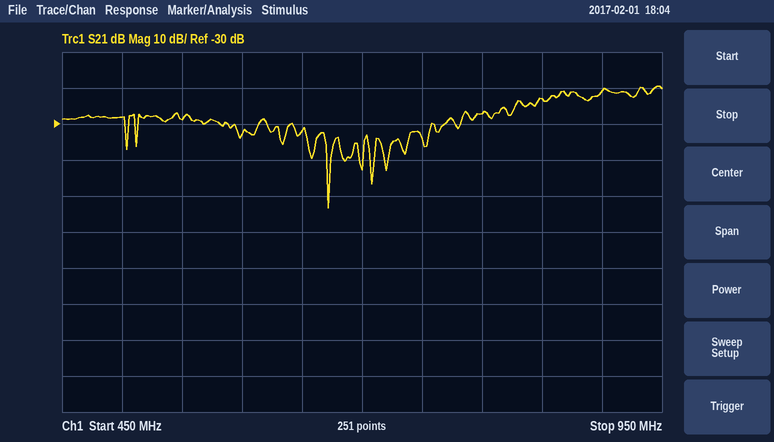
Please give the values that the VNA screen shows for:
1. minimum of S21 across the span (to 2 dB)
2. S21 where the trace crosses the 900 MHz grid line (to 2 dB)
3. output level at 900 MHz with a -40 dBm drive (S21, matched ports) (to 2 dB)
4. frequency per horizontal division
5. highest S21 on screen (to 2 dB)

-54 dB
-20 dB
-60 dBm
50 MHz
-20 dB
